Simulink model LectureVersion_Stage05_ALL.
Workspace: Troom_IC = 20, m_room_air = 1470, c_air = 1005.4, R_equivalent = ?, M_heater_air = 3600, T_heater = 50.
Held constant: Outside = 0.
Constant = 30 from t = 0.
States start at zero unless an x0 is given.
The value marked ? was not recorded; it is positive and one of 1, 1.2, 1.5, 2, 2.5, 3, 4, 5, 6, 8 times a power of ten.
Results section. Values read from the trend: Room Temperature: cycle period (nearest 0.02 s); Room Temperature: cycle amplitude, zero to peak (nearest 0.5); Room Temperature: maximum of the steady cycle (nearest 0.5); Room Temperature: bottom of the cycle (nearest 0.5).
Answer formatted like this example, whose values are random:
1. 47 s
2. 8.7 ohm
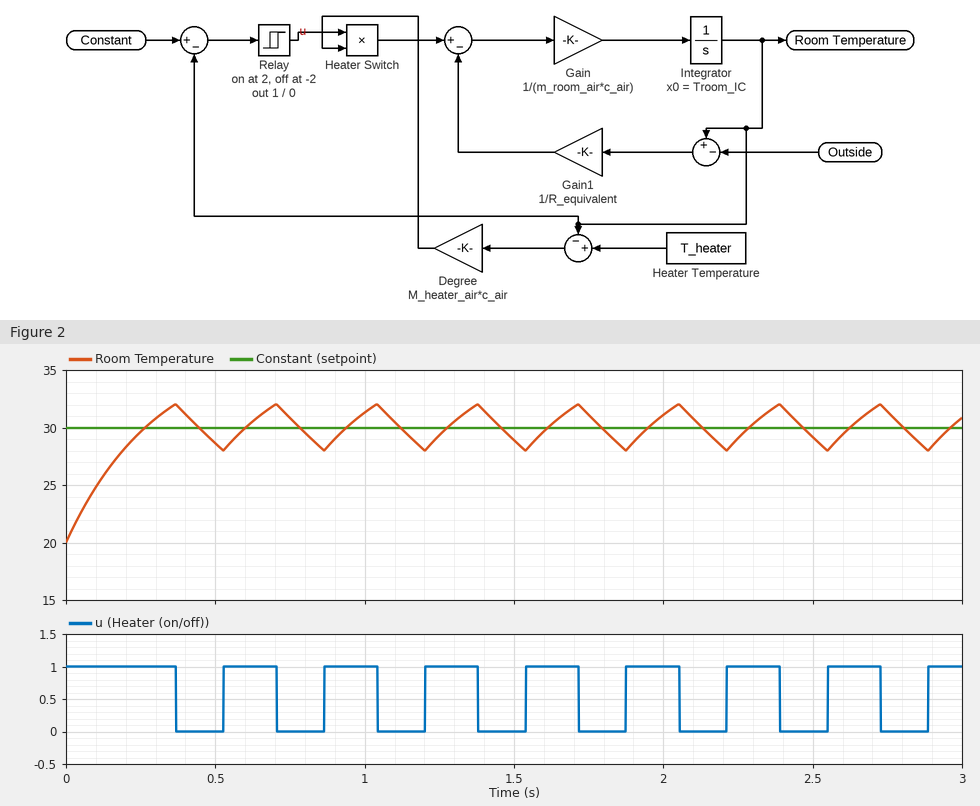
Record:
1. 0.34 s
2. 2.0
3. 32.0
4. 28.0
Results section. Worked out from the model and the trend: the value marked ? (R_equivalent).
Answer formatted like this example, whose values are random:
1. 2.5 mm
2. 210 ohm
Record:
1. 8e-07
